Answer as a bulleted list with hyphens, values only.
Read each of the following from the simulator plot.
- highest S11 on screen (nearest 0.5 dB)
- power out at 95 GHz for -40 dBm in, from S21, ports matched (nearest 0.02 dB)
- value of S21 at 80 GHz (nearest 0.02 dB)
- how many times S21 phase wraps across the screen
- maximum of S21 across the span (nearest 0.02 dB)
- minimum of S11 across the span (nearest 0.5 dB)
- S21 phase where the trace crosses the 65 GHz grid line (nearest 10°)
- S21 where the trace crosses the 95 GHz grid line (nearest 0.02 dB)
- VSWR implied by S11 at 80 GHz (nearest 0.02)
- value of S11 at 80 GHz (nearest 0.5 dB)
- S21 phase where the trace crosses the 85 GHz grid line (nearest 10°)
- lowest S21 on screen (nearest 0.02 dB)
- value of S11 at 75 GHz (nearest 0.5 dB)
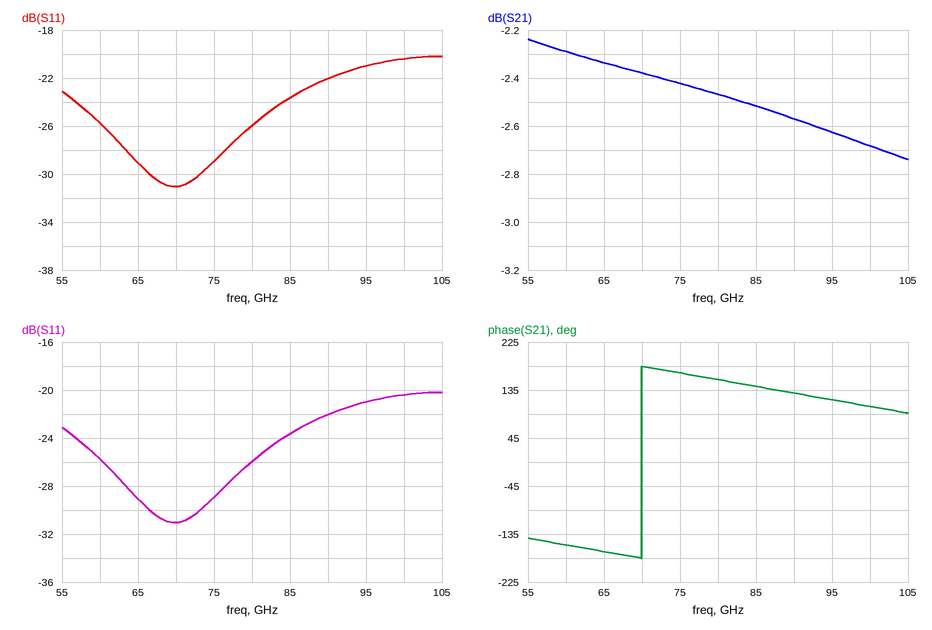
- -20.0 dB
- -42.62 dBm
- -2.46 dB
- 1
- -2.24 dB
- -31.0 dB
- -170°
- -2.62 dB
- 1.10
- -26.0 dB
- 140°
- -2.74 dB
- -29.0 dB
